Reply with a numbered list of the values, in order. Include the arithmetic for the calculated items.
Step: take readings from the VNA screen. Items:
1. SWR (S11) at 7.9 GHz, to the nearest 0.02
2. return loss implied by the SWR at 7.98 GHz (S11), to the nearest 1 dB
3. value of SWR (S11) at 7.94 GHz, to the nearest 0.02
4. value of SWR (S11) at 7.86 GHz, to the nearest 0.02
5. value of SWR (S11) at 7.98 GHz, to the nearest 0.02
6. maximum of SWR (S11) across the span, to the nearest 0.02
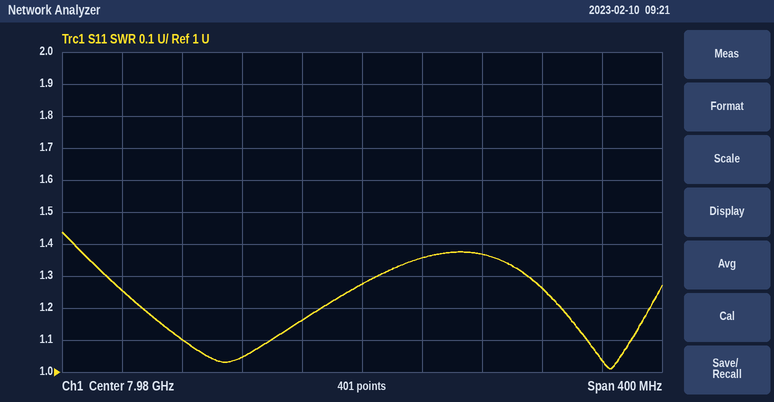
1. 1.04
2. −20 log10((1.28 − 1)/(1.28 + 1)) ≈ 18 dB
3. 1.16
4. 1.10
5. 1.28
6. 1.44
